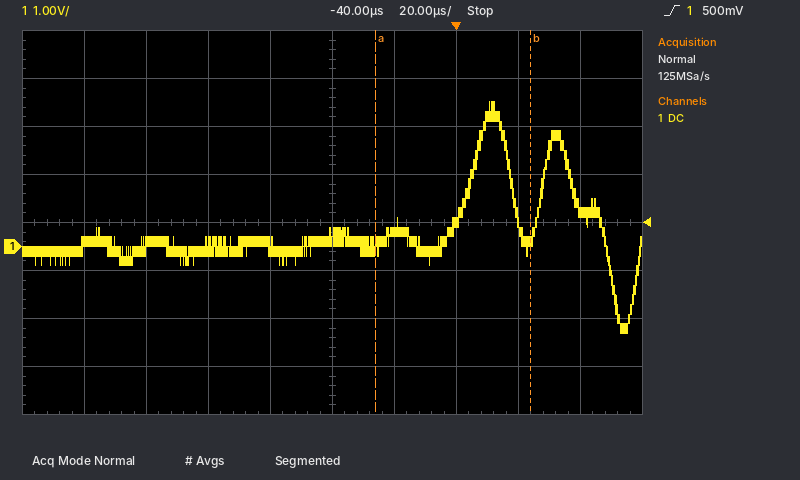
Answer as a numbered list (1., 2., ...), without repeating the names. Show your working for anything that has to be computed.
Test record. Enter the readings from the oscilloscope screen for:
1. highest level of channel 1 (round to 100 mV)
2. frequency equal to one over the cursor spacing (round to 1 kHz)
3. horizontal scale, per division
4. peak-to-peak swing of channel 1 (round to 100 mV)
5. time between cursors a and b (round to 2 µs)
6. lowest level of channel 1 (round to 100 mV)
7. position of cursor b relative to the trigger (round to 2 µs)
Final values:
1. 3.0 V
2. 1 / 50 µs ≈ 20 kHz
3. 20 µs
4. 3.0 V − (-1.8 V) = 4.8 V
5. 50 µs
6. -1.8 V
7. +24 µs
